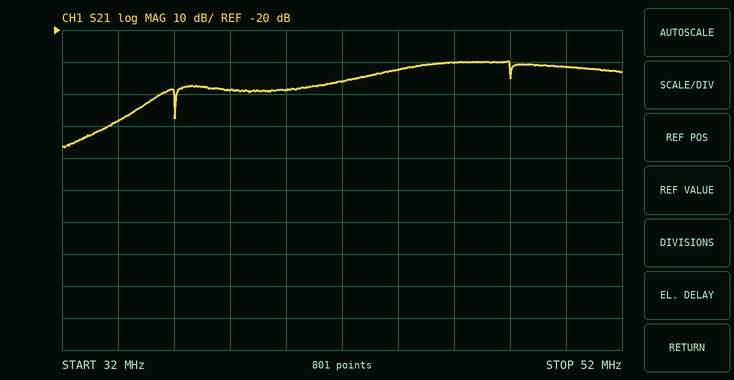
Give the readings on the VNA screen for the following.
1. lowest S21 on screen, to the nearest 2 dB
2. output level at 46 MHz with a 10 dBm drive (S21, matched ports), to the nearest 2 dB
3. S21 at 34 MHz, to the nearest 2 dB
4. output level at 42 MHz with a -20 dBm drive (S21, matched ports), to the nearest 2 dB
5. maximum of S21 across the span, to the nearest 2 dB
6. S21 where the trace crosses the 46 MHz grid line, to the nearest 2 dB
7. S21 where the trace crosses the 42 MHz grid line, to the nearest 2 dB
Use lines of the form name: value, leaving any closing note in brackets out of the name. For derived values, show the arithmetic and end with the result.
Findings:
lowest S21 on screen, to the nearest 2 dB: -56 dB
output level at 46 MHz with a 10 dBm drive (S21, matched ports), to the nearest 2 dB: 10 dBm + (-30 dB) = -20 dBm
S21 at 34 MHz, to the nearest 2 dB: -48 dB
output level at 42 MHz with a -20 dBm drive (S21, matched ports), to the nearest 2 dB: -20 dBm + (-36 dB) = -56 dBm
maximum of S21 across the span, to the nearest 2 dB: -30 dB
S21 where the trace crosses the 46 MHz grid line, to the nearest 2 dB: -30 dB
S21 where the trace crosses the 42 MHz grid line, to the nearest 2 dB: -36 dB
